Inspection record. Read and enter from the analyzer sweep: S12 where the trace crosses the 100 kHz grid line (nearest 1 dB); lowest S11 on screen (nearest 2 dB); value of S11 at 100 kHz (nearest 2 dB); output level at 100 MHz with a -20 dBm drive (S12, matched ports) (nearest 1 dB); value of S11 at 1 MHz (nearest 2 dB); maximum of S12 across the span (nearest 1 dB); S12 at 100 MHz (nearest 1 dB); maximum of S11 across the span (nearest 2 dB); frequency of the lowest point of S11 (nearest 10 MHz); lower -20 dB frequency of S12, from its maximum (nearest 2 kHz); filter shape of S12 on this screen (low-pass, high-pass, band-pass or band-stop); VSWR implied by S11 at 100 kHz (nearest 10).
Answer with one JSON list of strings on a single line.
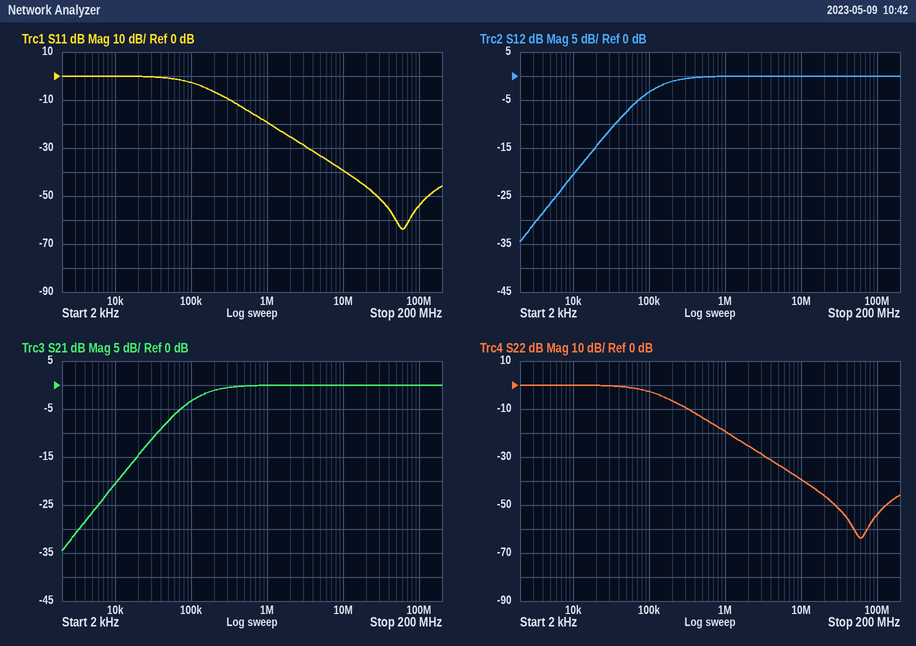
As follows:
["-3 dB", "-64 dB", "-2 dB", "-20 dBm", "-20 dB", "0 dB", "0 dB", "0 dB", "60 MHz", "10 kHz", "high-pass", "10"]
